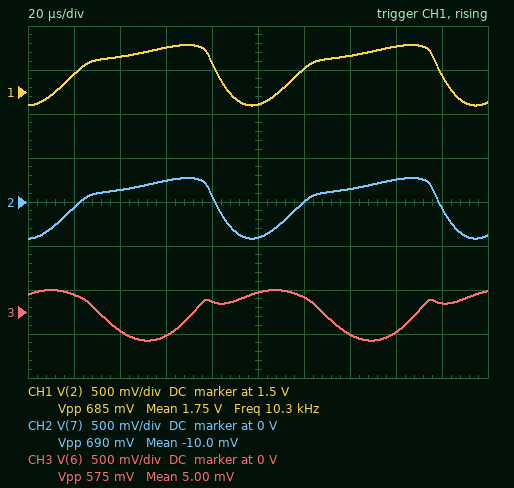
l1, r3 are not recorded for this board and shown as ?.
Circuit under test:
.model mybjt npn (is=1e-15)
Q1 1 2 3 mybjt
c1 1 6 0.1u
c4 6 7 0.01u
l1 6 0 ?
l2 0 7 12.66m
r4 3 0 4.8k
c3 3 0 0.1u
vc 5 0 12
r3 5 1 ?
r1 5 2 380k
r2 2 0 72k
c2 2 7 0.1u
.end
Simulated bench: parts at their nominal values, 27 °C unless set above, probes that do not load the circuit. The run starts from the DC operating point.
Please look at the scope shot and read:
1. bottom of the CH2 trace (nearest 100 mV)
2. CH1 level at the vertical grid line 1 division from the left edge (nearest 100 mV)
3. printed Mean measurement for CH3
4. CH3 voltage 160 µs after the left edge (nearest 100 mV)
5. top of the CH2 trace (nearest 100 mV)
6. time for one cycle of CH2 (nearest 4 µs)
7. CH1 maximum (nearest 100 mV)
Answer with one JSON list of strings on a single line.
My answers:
["-400 mV", "1.7 V", "5.00 mV", "-200 mV", "300 mV", "96 µs", "2.0 V"]
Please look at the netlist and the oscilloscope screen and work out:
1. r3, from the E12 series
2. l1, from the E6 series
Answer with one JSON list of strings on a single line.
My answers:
["680 Ω", "10 mH"]
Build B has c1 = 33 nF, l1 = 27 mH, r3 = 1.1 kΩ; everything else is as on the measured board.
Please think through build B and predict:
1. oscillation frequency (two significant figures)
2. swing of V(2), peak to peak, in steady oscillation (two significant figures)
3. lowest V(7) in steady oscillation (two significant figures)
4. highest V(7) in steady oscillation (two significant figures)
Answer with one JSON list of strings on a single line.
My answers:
["7.8 kHz", "470 mV", "-290 mV", "180 mV"]
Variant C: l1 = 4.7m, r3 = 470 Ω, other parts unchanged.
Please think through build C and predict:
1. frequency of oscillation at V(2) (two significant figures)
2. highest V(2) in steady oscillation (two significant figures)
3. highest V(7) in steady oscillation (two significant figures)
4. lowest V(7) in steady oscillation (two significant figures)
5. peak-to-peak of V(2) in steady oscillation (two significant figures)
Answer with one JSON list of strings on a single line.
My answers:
["12 kHz", "2.2 V", "460 mV", "-630 mV", "1.1 V"]
